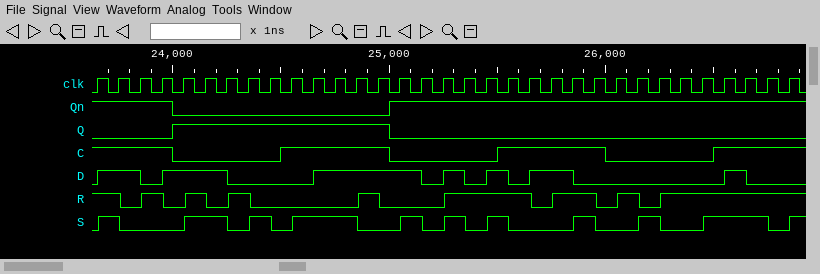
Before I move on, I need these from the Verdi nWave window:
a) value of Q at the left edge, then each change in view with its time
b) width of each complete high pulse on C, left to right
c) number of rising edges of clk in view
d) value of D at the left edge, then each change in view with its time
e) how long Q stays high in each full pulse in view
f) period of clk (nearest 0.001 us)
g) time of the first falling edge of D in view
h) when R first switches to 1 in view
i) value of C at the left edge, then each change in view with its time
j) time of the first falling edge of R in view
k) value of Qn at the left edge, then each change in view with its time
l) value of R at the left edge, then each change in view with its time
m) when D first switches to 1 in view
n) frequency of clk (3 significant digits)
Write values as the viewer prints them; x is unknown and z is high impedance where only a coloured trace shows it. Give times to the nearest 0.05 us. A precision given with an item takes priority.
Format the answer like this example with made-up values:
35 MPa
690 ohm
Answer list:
0, 1 at 24 us, 0 at 25 us
0.5 us, 0.5 us
33
0, 1 at 23.65 us, 0 at 23.85 us, 1 at 23.95 us, 0 at 24.25 us, 1 at 24.65 us, 0 at 25.15 us, 1 at 25.25 us, 0 at 25.35 us, 1 at 25.45 us, 0 at 25.55 us, 1 at 25.65 us, 0 at 25.85 us, 1 at 26.55 us, 0 at 26.65 us
1 us
0.1 us
23.85 us
23.85 us
1, 0 at 24 us, 1 at 24.5 us, 0 at 25 us, 1 at 25.5 us, 0 at 26 us, 1 at 26.5 us
23.75 us
1, 0 at 24 us, 1 at 25 us
1, 0 at 23.75 us, 1 at 23.85 us, 0 at 23.95 us, 1 at 24.05 us, 0 at 24.15 us, 1 at 24.25 us, 0 at 24.35 us, 1 at 24.85 us, 0 at 24.95 us, 1 at 25.25 us, 0 at 25.65 us, 1 at 25.75 us, 0 at 25.95 us, 1 at 26.05 us, 0 at 26.15 us, 1 at 26.25 us
23.65 us
10.0 MHz
